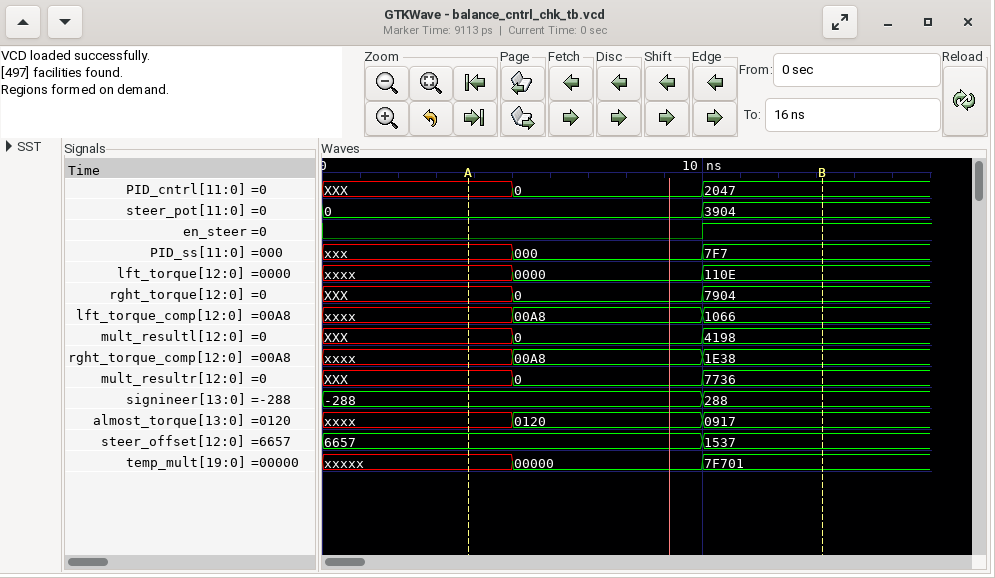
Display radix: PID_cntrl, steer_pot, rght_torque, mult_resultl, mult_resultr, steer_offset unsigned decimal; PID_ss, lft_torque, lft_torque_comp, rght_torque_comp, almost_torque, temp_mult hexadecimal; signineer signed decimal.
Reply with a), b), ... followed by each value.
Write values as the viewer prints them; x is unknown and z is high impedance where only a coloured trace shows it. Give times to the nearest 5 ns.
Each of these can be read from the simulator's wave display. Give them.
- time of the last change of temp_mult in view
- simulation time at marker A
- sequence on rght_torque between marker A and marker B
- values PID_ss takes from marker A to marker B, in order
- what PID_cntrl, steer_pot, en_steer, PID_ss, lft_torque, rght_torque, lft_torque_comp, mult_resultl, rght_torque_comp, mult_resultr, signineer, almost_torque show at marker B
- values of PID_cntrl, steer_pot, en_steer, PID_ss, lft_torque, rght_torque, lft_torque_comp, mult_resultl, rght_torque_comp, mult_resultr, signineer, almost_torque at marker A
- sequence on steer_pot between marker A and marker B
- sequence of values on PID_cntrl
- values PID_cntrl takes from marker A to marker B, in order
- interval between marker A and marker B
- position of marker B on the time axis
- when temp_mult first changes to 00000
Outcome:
a) 10 ns
b) 5 ns
c) XXX, 0, 7904
d) xxx, 000, 7F7
e) PID_cntrl=2047, steer_pot=3904, en_steer=1, PID_ss=7F7, lft_torque=110E, rght_torque=7904, lft_torque_comp=1066, mult_resultl=4198, rght_torque_comp=1E38, mult_resultr=7736, signineer=288, almost_torque=0917
f) PID_cntrl=XXX, steer_pot=0, en_steer=0, PID_ss=xxx, lft_torque=xxxx, rght_torque=XXX, lft_torque_comp=xxxx, mult_resultl=XXX, rght_torque_comp=xxxx, mult_resultr=XXX, signineer=-288, almost_torque=xxxx
g) 0, 3904
h) XXX, 0, 2047
i) XXX, 0, 2047
j) 10 ns
k) 15 ns
l) 5 ns
